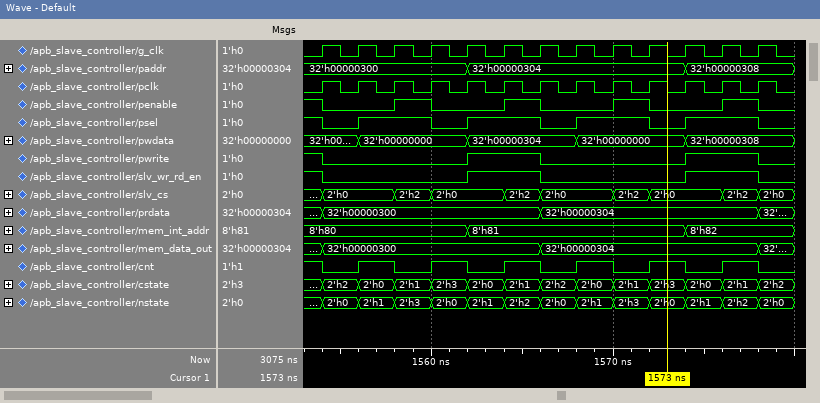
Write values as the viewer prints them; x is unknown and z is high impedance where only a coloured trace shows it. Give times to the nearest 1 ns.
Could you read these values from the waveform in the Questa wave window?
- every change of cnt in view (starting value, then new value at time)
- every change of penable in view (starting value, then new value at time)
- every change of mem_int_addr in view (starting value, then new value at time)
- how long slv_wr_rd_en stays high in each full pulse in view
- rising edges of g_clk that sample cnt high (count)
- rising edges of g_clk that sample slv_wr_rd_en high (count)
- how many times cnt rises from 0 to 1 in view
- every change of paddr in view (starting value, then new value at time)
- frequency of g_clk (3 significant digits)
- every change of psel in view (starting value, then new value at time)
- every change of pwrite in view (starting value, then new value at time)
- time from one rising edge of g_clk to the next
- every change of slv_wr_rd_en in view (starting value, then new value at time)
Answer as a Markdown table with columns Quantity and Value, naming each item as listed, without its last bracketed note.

| Quantity | Value |
|---|---|
| every change of cnt in view | 1, 0 at 1554 ns, 1 at 1556 ns, 0 at 1558 ns, 1 at 1560 ns, 0 at 1562 ns, 1 at 1564 ns, 0 at 1566 ns, 1 at 1568 ns, 0 at 1570 ns, 1 at 1572 ns, 0 at 1574 ns, 1 at 1576 ns, 0 at 1578 ns |
| every change of penable in view | 1, 0 at 1554 ns, 1 at 1558 ns, 0 at 1560 ns, 1 at 1564 ns, 0 at 1566 ns, 1 at 1570 ns, 0 at 1572 ns, 1 at 1576 ns, 0 at 1578 ns |
| every change of mem_int_addr in view | 8'h80, 8'h81 at 1562 ns, 8'h82 at 1574 ns |
| how long slv_wr_rd_en stays high in each full pulse in view | 4 ns, 4 ns |
| rising edges of g_clk that sample cnt high | 7 |
| rising edges of g_clk that sample slv_wr_rd_en high | 5 |
| how many times cnt rises from 0 to 1 in view | 6 |
| every change of paddr in view | 32'h00000300, 32'h00000304 at 1562 ns, 32'h00000308 at 1574 ns |
| frequency of g_clk | 500 MHz |
| every change of psel in view | 1, 0 at 1554 ns, 1 at 1556 ns, 0 at 1560 ns, 1 at 1562 ns, 0 at 1566 ns, 1 at 1568 ns, 0 at 1572 ns, 1 at 1574 ns, 0 at 1578 ns |
| every change of pwrite in view | 1, 0 at 1554 ns, 1 at 1562 ns, 0 at 1566 ns, 1 at 1574 ns, 0 at 1578 ns |
| time from one rising edge of g_clk to the next | 2 ns |
| every change of slv_wr_rd_en in view | 1, 0 at 1554 ns, 1 at 1562 ns, 0 at 1566 ns, 1 at 1574 ns, 0 at 1578 ns |
